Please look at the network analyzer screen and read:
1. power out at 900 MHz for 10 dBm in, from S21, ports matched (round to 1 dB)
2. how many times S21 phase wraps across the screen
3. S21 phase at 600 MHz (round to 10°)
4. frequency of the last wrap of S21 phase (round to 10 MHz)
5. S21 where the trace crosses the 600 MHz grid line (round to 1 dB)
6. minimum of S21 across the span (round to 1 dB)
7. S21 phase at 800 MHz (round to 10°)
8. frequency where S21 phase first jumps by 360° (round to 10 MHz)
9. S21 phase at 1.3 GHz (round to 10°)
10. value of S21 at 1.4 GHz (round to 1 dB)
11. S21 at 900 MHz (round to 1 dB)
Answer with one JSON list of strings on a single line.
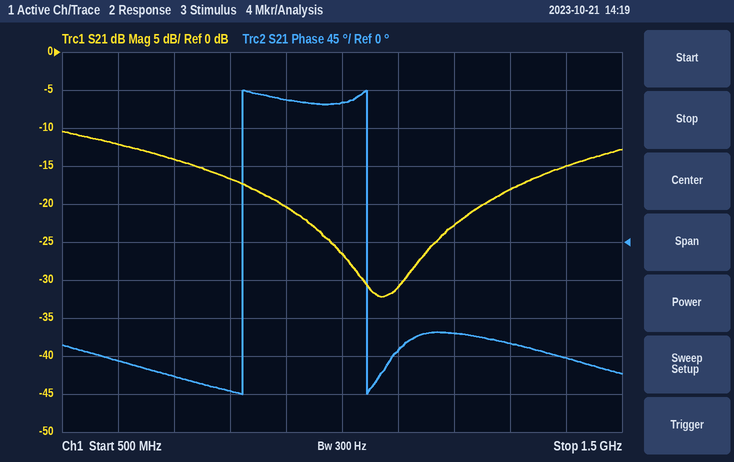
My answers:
["-10 dBm", "2", "-140°", "1.04 GHz", "-12 dB", "-32 dB", "-180°", "820 MHz", "-120°", "-15 dB", "-20 dB"]
